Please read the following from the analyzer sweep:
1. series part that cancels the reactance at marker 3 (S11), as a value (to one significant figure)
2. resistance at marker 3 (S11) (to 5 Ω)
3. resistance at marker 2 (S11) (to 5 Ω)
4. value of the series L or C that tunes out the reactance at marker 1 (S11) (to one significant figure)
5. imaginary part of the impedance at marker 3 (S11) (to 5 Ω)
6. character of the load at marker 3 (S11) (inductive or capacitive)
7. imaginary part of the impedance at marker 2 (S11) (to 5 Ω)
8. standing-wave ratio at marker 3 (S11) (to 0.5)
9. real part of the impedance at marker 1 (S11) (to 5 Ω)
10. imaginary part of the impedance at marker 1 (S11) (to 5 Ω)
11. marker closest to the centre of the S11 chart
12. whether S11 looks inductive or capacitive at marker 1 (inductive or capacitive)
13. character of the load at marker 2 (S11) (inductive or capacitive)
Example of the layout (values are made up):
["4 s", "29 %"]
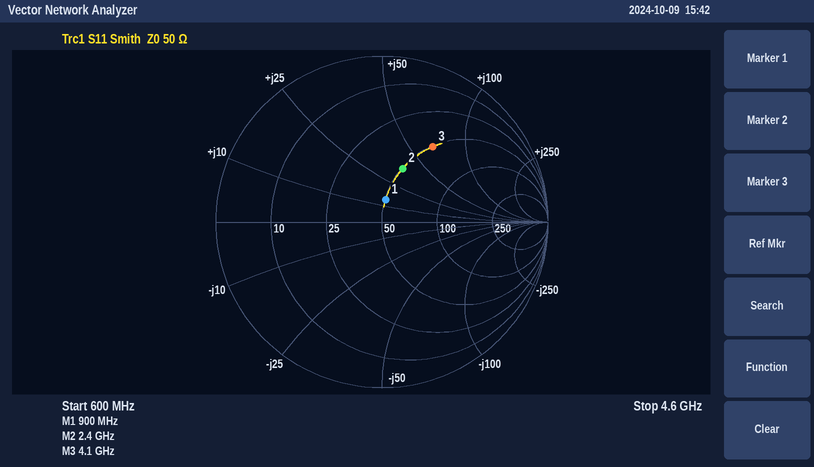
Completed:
["600 fF", "50 Ω", "50 Ω", "10 pF", "+65 Ω", "inductive", "+35 Ω", "3.5", "50 Ω", "+15 Ω", "marker 1", "inductive", "inductive"]
